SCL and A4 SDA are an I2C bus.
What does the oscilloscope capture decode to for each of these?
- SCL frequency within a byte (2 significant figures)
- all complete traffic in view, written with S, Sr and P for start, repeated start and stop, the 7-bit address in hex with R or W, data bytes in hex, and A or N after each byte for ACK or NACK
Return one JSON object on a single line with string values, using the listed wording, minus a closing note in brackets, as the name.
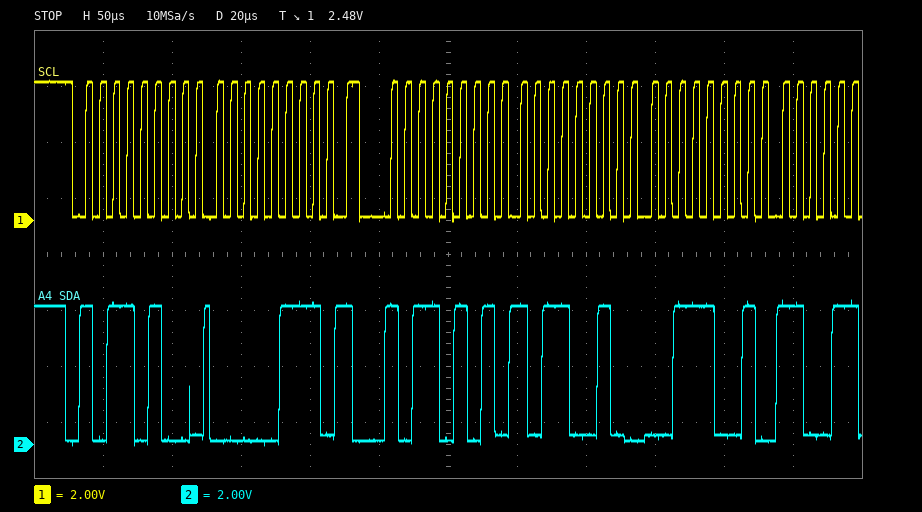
{"SCL frequency within a byte": "100 kHz", "all complete traffic in view, written with S, Sr and P for start, repeated start and stop, the 7-bit address in hex with R or W, data bytes in hex, and A or N after each byte for ACK or NACK": "S 5AW A 07 A Sr 5AR A B2 A 39 A"}
